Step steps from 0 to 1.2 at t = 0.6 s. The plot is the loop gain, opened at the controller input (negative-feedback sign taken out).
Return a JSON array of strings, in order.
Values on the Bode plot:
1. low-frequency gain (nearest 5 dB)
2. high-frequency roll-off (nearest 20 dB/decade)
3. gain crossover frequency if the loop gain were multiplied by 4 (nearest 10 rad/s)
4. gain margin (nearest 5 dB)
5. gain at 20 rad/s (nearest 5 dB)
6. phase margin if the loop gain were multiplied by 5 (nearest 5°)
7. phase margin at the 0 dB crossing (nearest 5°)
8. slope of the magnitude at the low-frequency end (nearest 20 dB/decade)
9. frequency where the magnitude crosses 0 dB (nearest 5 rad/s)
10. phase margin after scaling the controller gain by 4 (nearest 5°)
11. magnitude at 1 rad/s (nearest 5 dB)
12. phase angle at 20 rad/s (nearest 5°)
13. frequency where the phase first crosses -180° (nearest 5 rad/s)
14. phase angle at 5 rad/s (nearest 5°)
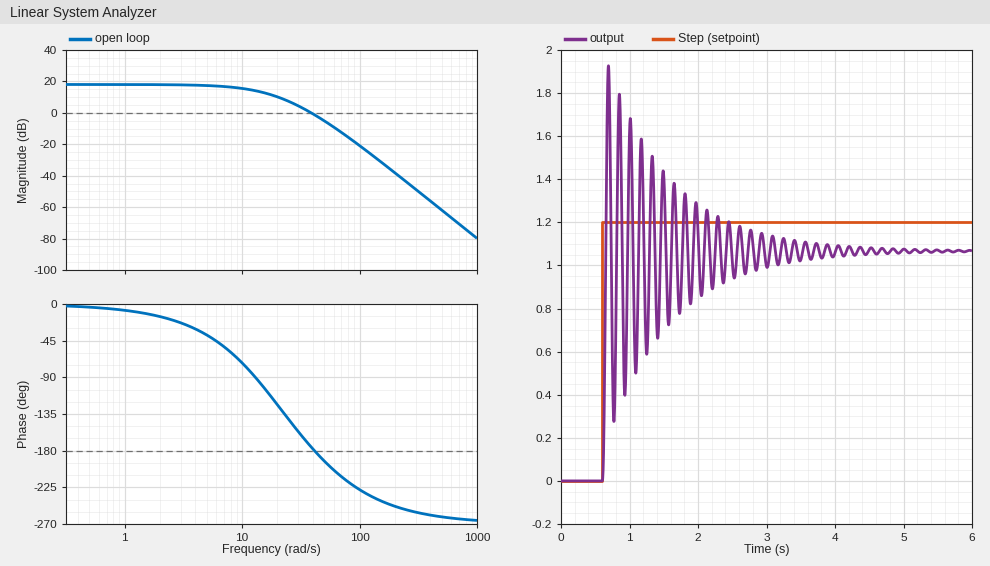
["20 dB", "-60 dB/decade", "70 rad/s", "0 dB", "10 dB", "-35°", "5°", "0 dB/decade", "40 rad/s", "-30°", "20 dB", "-125°", "40 rad/s", "-40°"]
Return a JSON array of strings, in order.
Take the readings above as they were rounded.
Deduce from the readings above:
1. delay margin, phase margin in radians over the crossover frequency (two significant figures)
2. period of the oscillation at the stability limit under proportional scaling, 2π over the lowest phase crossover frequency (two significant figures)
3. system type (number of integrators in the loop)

["0.0022 s", "0.16 s", "0"]
